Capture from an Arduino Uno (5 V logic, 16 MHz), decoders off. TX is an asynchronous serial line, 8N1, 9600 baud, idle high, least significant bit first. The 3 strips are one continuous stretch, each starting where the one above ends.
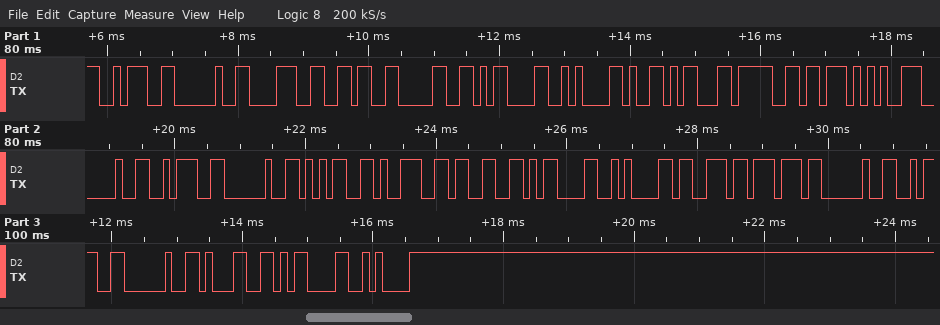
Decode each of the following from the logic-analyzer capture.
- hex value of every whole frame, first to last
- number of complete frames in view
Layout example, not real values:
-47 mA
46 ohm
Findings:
0x3A 0x20 0x38 0x36 0x30 0x0D 0x0A 0x59 0xEC 0xB6 0x95 0x20 0x3A 0x20 0x35 0x39 0x33 0x0D 0x0A 0x73 0x77 0x20 0x3A 0x20 0x31 0x0D 0x0A
27
